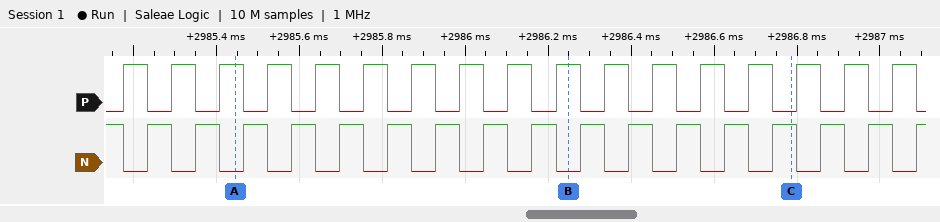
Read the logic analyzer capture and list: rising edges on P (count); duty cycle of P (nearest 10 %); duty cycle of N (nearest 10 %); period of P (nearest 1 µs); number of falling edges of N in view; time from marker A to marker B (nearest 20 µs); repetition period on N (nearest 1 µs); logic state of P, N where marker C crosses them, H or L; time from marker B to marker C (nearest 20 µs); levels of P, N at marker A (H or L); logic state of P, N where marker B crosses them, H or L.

17
50 %
50 %
116 µs
17
800 µs
116 µs
P=L, N=H
540 µs
P=H, N=L
P=H, N=L
